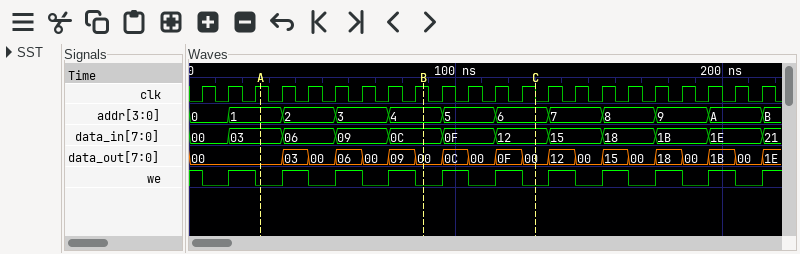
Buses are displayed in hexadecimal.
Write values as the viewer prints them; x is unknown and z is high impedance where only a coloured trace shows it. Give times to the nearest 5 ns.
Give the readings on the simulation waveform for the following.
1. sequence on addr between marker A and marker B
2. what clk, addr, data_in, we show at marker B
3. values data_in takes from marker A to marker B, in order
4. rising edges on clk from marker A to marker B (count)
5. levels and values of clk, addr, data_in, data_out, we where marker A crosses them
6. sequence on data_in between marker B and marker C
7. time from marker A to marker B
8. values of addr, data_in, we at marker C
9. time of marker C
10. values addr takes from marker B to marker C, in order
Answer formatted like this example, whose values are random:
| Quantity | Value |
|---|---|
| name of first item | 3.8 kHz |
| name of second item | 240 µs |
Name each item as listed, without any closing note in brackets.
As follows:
| Quantity | Value |
|---|---|
| sequence on addr between marker A and marker B | 1, 2, 3, 4 |
| what clk, addr, data_in, we show at marker B | clk=1, addr=4, data_in=0C, we=0 |
| values data_in takes from marker A to marker B, in order | 03, 06, 09, 0C |
| rising edges on clk from marker A to marker B | 6 |
| levels and values of clk, addr, data_in, data_out, we where marker A crosses them | clk=1, addr=1, data_in=03, data_out=00, we=0 |
| sequence on data_in between marker B and marker C | 0C, 0F, 12 |
| time from marker A to marker B | 60 ns |
| values of addr, data_in, we at marker C | addr=6, data_in=12, we=0 |
| time of marker C | 130 ns |
| values addr takes from marker B to marker C, in order | 4, 5, 6 |
